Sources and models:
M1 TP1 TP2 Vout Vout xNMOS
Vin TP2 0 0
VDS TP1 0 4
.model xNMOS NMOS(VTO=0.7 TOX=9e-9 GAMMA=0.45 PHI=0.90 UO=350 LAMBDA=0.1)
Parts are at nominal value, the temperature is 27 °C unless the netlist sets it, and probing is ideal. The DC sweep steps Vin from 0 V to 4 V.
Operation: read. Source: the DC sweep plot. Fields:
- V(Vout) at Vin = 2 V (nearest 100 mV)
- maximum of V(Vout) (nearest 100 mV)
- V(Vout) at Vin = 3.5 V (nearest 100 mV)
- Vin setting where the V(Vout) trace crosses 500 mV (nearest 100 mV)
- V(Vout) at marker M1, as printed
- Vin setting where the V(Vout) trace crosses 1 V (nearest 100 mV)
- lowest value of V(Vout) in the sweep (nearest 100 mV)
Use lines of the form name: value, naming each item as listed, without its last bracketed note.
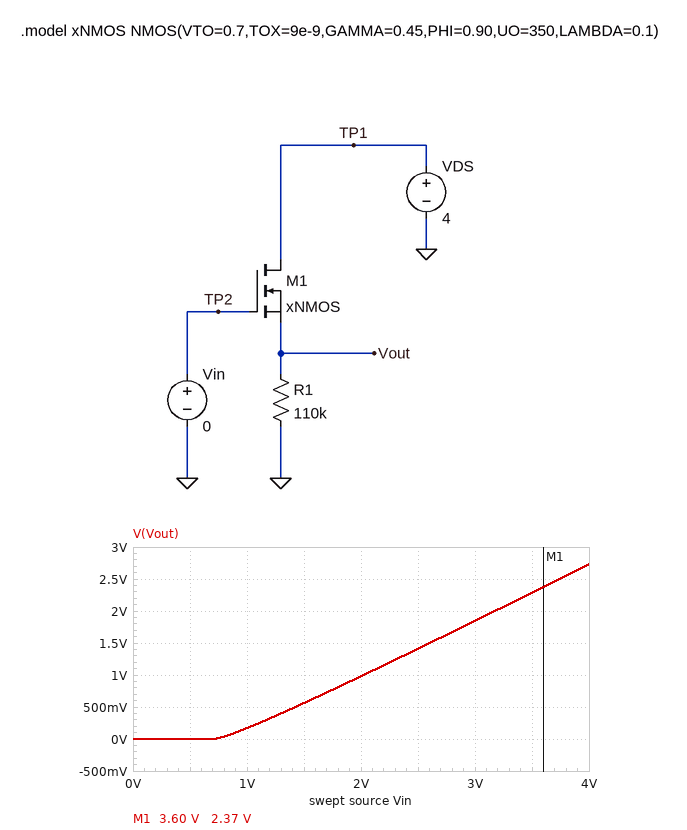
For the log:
V(Vout) at Vin = 2 V: 1.0 V
maximum of V(Vout): 2.7 V
V(Vout) at Vin = 3.5 V: 2.3 V
Vin setting where the V(Vout) trace crosses 500 mV: 1.4 V
V(Vout) at marker M1, as printed: 2.37 V
Vin setting where the V(Vout) trace crosses 1 V: 2.0 V
lowest value of V(Vout) in the sweep: 0 V
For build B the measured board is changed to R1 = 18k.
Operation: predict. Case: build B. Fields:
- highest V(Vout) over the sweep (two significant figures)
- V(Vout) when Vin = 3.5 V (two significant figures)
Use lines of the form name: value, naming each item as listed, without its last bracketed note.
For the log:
highest V(Vout) over the sweep: 2.1 V
V(Vout) when Vin = 3.5 V: 1.7 V
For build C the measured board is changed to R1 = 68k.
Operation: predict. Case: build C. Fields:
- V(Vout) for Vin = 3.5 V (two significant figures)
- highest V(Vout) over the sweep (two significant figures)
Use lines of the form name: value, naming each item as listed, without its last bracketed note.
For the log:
V(Vout) for Vin = 3.5 V: 2.2 V
highest V(Vout) over the sweep: 2.6 V
